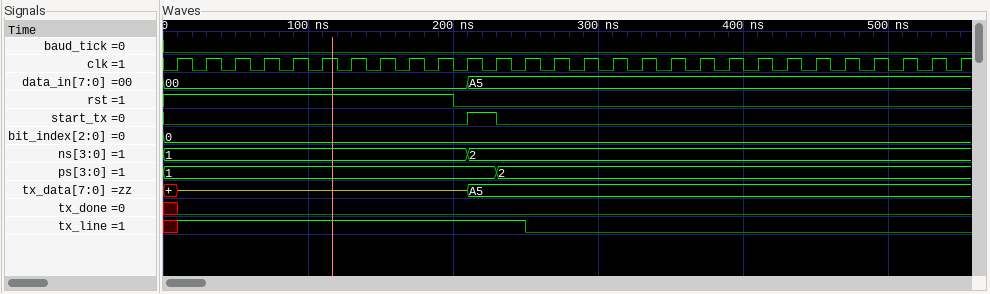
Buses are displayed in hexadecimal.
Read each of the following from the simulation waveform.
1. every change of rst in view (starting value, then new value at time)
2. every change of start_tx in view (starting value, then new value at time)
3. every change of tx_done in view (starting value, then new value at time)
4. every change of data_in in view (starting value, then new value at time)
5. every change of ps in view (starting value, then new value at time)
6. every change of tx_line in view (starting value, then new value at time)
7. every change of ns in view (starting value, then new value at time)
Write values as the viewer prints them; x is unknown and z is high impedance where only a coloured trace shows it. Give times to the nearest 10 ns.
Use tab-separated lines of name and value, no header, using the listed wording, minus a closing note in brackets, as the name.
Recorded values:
every change of rst in view	1, 0 at 200 ns
every change of start_tx in view	0, 1 at 210 ns, 0 at 230 ns
every change of tx_done in view	x, 0 at 10 ns
every change of data_in in view	00, A5 at 210 ns
every change of ps in view	1, 2 at 230 ns
every change of tx_line in view	x, 1 at 10 ns, 0 at 250 ns
every change of ns in view	1, 2 at 210 ns
